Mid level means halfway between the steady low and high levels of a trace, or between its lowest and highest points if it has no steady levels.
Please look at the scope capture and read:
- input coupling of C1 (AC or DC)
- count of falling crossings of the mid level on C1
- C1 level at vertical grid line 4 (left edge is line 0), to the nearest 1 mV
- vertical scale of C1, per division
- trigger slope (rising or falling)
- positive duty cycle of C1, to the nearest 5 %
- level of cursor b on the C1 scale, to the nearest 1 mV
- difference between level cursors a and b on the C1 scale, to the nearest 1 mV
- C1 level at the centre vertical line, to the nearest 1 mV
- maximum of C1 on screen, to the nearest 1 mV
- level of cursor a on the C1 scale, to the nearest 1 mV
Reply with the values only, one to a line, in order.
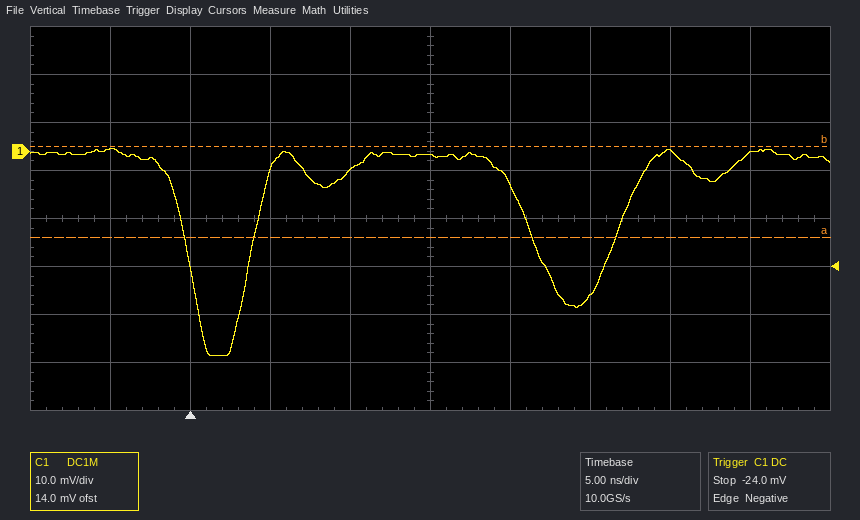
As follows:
DC
2
-4 mV
10 mV
falling
80 %
1 mV
19 mV
-1 mV
1 mV
-18 mV
